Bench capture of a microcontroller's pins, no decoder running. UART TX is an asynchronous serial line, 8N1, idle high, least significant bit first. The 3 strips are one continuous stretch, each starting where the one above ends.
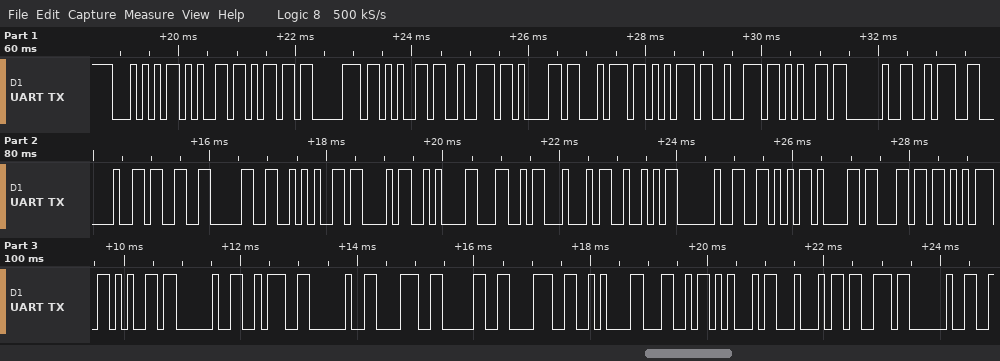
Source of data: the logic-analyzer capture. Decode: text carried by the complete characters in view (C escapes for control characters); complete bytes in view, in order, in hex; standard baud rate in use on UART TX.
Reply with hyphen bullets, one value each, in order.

- "Temperature : 30*C\nLDR Value : 808\nLEDs "
- 54 65 6D 70 65 72 61 74 75 72 65 20 3A 20 33 30 2A 43 0A 4C 44 52 20 56 61 6C 75 65 20 3A 20 38 30 38 0A 4C 45 44 73 20
- 9600 baud
